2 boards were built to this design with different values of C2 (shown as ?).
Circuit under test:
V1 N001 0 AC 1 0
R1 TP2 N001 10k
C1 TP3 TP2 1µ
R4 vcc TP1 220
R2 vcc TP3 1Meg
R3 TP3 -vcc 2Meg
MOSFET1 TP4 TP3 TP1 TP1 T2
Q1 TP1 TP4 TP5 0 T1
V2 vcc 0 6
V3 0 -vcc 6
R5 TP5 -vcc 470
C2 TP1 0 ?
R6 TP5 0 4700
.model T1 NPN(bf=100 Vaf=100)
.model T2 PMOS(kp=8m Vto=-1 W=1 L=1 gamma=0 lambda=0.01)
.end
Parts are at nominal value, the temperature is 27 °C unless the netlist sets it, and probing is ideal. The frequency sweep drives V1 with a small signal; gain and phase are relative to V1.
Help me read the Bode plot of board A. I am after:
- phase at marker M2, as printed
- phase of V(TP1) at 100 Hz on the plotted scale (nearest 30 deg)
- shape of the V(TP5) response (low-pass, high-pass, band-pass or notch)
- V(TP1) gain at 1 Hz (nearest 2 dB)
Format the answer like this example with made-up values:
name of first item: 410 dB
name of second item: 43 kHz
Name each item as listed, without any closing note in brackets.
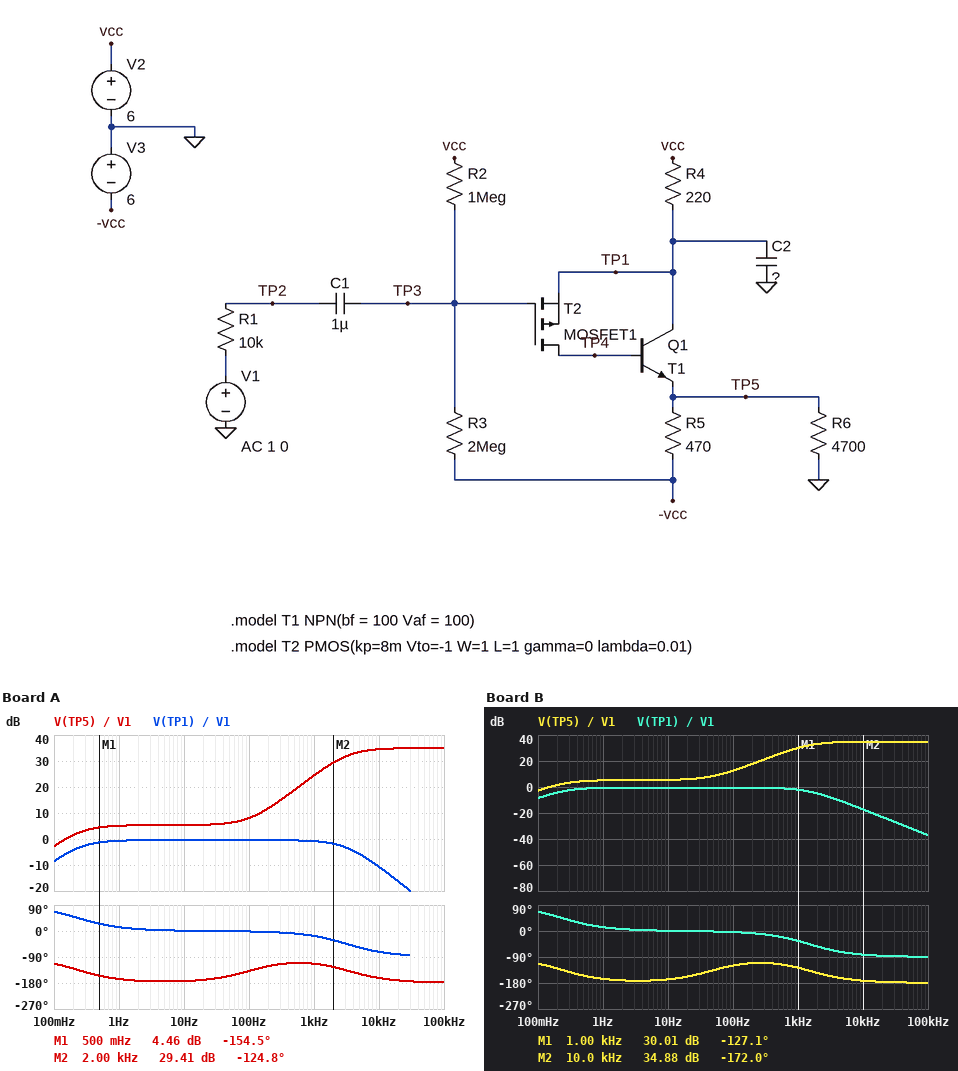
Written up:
phase at marker M2, as printed: -124.8 deg
phase of V(TP1) at 100 Hz on the plotted scale: 0 deg
shape of the V(TP5) response: high-pass
V(TP1) gain at 1 Hz: 0 dB
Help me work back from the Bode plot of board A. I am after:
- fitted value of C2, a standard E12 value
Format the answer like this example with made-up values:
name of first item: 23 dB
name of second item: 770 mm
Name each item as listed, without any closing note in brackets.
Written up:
fitted value of C2, a standard E12 value: 6.8 µF
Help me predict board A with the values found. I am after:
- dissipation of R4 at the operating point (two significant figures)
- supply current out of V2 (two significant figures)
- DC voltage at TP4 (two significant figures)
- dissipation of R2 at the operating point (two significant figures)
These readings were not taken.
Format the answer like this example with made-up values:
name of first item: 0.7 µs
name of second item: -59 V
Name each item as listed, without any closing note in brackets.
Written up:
dissipation of R4 at the operating point: 36 mW
supply current out of V2: 13 mA
DC voltage at TP4: 870 mV
dissipation of R2 at the operating point: 16 µW
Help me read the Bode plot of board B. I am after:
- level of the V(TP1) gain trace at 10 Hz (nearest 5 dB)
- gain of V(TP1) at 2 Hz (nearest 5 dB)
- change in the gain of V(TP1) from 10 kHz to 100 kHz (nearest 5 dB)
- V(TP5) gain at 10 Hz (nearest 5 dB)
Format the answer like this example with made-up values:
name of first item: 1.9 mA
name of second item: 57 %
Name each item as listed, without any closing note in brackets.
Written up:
level of the V(TP1) gain trace at 10 Hz: 0 dB
gain of V(TP1) at 2 Hz: 0 dB
change in the gain of V(TP1) from 10 kHz to 100 kHz: -20 dB
V(TP5) gain at 10 Hz: 5 dB
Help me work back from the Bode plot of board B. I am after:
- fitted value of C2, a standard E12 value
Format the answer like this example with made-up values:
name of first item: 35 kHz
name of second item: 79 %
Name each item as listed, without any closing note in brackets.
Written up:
fitted value of C2, a standard E12 value: 15 µF
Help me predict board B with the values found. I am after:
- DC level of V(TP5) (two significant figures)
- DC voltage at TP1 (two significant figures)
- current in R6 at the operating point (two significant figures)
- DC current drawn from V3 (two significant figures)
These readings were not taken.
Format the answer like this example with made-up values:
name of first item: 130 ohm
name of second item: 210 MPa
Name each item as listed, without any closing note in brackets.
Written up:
DC level of V(TP5): 33 mV
DC voltage at TP1: 3.2 V
current in R6 at the operating point: 7.1 µA
DC current drawn from V3: 13 mA
